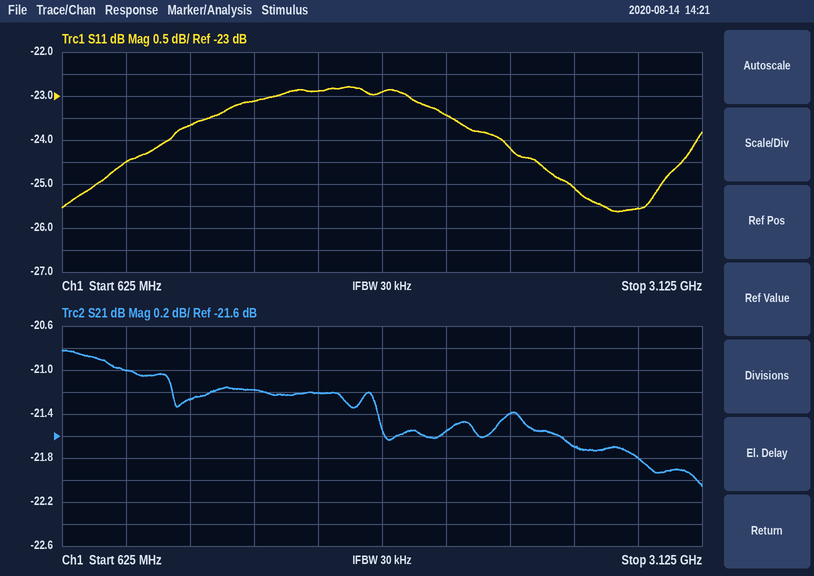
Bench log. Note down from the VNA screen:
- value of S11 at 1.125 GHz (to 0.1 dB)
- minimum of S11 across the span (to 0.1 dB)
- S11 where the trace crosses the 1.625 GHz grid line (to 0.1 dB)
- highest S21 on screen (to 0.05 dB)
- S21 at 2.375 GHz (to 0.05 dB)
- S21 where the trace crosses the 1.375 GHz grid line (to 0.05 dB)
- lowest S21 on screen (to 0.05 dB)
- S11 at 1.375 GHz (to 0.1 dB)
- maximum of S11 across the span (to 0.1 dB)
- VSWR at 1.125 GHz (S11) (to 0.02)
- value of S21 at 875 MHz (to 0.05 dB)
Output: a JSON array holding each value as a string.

["-23.7 dB", "-25.6 dB", "-22.9 dB", "-20.80 dB", "-21.40 dB", "-21.20 dB", "-22.05 dB", "-23.1 dB", "-22.8 dB", "1.14", "-21.00 dB"]
